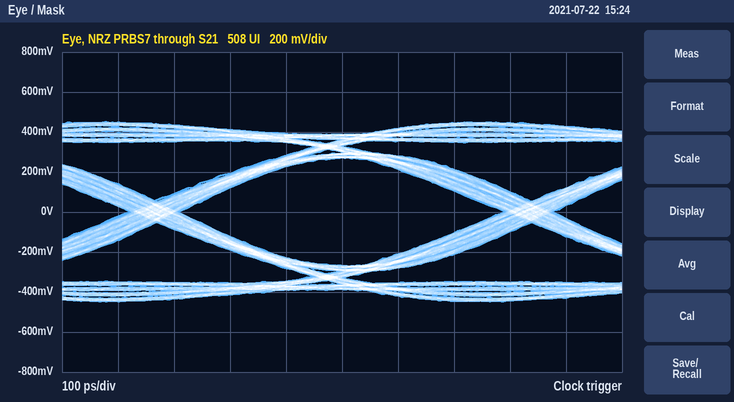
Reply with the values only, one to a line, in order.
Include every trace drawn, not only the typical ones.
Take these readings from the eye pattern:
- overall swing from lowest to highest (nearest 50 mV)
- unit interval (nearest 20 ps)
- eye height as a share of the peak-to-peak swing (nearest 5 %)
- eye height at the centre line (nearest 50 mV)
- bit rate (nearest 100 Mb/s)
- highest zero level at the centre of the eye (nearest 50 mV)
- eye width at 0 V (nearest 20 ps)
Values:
900 mV
660 ps
60 %
550 mV
1.5 Gb/s
-250 mV
580 ps
